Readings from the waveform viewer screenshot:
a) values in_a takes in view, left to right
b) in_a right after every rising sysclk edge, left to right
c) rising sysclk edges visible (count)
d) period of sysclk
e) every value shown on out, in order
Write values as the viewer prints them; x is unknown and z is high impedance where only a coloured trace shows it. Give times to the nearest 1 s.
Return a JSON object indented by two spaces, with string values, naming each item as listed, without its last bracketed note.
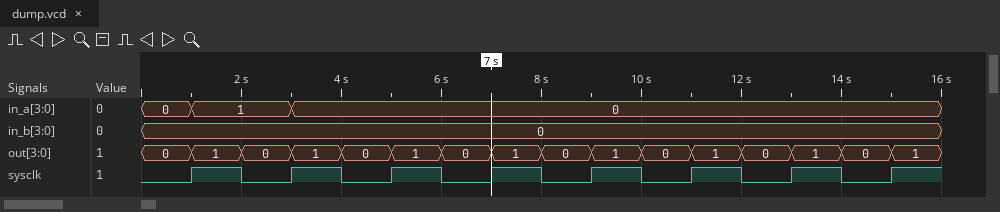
{
  "values in_a takes in view, left to right": "0, 1, 0",
  "in_a right after every rising sysclk edge, left to right": "1, 0, 0, 0, 0, 0, 0, 0",
  "rising sysclk edges visible": "8",
  "period of sysclk": "2 s",
  "every value shown on out, in order": "0, 1, 0, 1, 0, 1, 0, 1, 0, 1, 0, 1, 0, 1, 0, 1"
}
